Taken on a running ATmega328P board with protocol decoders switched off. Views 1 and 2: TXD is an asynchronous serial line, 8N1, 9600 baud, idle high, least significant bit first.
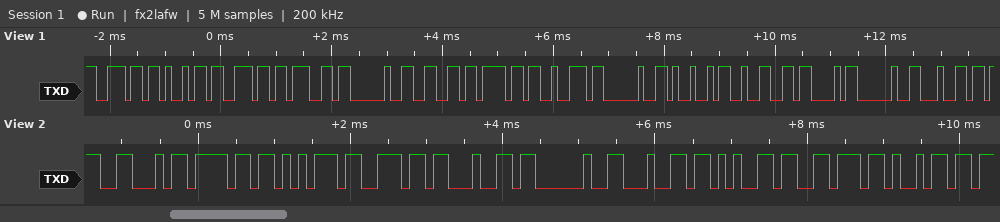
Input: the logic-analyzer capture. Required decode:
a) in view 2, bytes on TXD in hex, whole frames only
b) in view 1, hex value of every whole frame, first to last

46 6F 75 6E 64 20 64 65 76 69
0x6E 0x69 0x6E 0x67 0x20 0x66 0x6F 0x72 0x20 0x49 0x32 0x43 0x20 0x64
